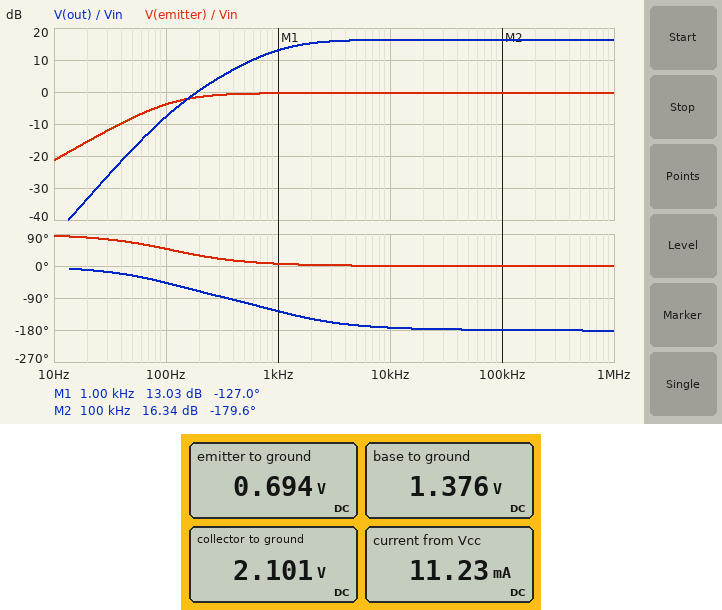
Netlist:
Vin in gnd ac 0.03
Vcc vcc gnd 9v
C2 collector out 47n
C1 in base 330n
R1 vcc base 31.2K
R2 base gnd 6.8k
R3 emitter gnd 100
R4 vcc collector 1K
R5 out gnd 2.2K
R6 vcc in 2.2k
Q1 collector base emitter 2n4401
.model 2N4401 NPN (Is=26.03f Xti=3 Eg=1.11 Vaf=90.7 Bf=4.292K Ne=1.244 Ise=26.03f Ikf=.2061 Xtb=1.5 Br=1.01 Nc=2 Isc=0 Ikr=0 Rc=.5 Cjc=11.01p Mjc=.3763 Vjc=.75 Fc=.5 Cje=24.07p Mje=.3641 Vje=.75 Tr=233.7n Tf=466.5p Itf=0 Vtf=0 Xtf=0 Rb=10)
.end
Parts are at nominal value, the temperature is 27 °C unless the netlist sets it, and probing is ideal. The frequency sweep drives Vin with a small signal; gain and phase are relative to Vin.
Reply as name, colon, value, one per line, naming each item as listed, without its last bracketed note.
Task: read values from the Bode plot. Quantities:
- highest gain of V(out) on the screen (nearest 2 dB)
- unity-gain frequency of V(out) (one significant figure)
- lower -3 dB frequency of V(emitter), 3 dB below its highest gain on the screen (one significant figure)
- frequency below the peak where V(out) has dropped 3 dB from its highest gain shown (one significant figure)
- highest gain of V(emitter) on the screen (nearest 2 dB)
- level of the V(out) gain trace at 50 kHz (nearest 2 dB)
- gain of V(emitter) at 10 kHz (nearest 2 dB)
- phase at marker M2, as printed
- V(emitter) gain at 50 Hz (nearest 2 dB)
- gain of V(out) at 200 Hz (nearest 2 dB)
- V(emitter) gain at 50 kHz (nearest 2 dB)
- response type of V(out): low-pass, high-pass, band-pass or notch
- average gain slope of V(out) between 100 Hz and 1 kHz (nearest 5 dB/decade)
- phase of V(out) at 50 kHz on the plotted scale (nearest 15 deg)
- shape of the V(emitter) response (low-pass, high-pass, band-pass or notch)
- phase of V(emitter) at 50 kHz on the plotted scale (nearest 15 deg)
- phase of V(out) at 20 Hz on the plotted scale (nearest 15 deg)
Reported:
highest gain of V(out) on the screen: 16 dB
unity-gain frequency of V(out): 200 Hz
lower -3 dB frequency of V(emitter), 3 dB below its highest gain on the screen: 100 Hz
frequency below the peak where V(out) has dropped 3 dB from its highest gain shown: 1 kHz
highest gain of V(emitter) on the screen: 0 dB
level of the V(out) gain trace at 50 kHz: 16 dB
gain of V(emitter) at 10 kHz: 0 dB
phase at marker M2, as printed: -179.6 deg
V(emitter) gain at 50 Hz: -8 dB
gain of V(out) at 200 Hz: 0 dB
V(emitter) gain at 50 kHz: 0 dB
response type of V(out): low-pass, high-pass, band-pass or notch: high-pass
average gain slope of V(out) between 100 Hz and 1 kHz: 20 dB/decade
phase of V(out) at 50 kHz on the plotted scale: -180 deg
shape of the V(emitter) response: high-pass
phase of V(emitter) at 50 kHz on the plotted scale: 0 deg
phase of V(out) at 20 Hz on the plotted scale: -15 deg
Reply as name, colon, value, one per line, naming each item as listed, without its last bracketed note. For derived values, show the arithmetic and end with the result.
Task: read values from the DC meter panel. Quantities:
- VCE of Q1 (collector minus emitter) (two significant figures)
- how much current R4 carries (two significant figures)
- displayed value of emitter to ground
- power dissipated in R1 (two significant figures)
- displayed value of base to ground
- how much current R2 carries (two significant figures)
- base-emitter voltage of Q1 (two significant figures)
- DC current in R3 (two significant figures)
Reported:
VCE of Q1 (collector minus emitter): 2.101 V - 694 mV = 1.4 V
how much current R4 carries: (9 V - 2.101 V) / 1 kΩ = 6.9 mA
displayed value of emitter to ground: 0.694 V
power dissipated in R1: (9 V - 1.376 V)^2 / 31.2 kΩ = 1.9 mW
displayed value of base to ground: 1.376 V
how much current R2 carries: (1.376 V) / 6.8 kΩ = 200 µA
base-emitter voltage of Q1: 1.376 V - 694 mV = 680 mV
DC current in R3: (694 mV) / 100 Ω = 6.9 mA
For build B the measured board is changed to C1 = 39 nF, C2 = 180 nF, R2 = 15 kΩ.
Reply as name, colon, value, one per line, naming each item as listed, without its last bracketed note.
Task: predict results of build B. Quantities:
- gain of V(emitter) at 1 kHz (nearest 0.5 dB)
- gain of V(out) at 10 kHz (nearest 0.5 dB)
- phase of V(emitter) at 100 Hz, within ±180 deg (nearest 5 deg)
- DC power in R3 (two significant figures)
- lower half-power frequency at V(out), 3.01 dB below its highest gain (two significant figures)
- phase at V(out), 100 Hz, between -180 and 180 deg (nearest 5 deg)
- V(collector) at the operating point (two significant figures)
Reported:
gain of V(emitter) at 1 kHz: -30.5 dB
gain of V(out) at 10 kHz: -9.0 dB
phase of V(emitter) at 100 Hz, within ±180 deg: 90 deg
DC power in R3: 6.7 mW
lower half-power frequency at V(out), 3.01 dB below its highest gain: 28 kHz
phase at V(out), 100 Hz, between -180 and 180 deg: -15 deg
V(collector) at the operating point: 940 mV
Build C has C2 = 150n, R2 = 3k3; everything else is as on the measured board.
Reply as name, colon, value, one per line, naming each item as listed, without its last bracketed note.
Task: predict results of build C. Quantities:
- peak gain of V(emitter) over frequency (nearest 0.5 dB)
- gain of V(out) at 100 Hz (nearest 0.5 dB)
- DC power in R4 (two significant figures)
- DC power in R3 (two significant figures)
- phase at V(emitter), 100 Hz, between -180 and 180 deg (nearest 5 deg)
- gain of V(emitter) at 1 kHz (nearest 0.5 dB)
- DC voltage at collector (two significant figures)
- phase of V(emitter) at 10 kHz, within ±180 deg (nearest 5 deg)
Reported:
peak gain of V(emitter) over frequency: -1.0 dB
gain of V(out) at 100 Hz: -2.0 dB
DC power in R4: 3.1 mW
DC power in R3: 320 µW
phase at V(emitter), 100 Hz, between -180 and 180 deg: 60 deg
gain of V(emitter) at 1 kHz: -1.5 dB
DC voltage at collector: 7.2 V
phase of V(emitter) at 10 kHz, within ±180 deg: 0 deg
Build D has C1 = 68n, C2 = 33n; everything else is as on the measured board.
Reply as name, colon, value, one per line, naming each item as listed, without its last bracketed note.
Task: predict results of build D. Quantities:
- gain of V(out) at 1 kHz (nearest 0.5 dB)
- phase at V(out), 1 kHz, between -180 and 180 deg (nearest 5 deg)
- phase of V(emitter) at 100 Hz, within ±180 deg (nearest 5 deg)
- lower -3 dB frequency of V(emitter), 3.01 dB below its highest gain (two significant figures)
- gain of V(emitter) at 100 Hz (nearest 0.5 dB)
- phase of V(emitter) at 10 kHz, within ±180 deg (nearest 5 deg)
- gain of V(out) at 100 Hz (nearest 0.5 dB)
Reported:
gain of V(out) at 1 kHz: 10.0 dB
phase at V(out), 1 kHz, between -180 and 180 deg: -95 deg
phase of V(emitter) at 100 Hz, within ±180 deg: 80 deg
lower -3 dB frequency of V(emitter), 3.01 dB below its highest gain: 540 Hz
gain of V(emitter) at 100 Hz: -15.0 dB
phase of V(emitter) at 10 kHz, within ±180 deg: 5 deg
gain of V(out) at 100 Hz: -22.0 dB
